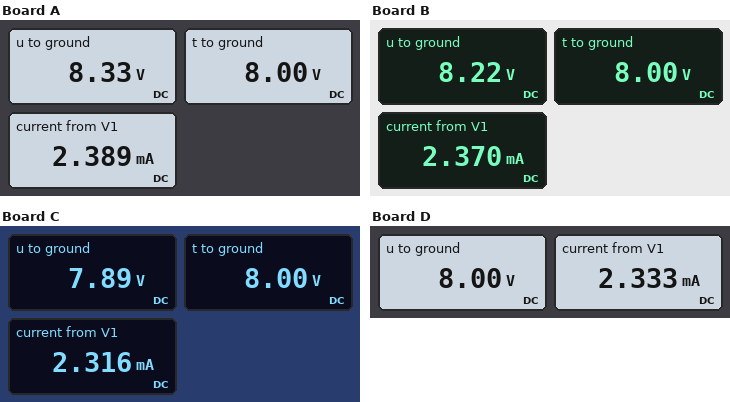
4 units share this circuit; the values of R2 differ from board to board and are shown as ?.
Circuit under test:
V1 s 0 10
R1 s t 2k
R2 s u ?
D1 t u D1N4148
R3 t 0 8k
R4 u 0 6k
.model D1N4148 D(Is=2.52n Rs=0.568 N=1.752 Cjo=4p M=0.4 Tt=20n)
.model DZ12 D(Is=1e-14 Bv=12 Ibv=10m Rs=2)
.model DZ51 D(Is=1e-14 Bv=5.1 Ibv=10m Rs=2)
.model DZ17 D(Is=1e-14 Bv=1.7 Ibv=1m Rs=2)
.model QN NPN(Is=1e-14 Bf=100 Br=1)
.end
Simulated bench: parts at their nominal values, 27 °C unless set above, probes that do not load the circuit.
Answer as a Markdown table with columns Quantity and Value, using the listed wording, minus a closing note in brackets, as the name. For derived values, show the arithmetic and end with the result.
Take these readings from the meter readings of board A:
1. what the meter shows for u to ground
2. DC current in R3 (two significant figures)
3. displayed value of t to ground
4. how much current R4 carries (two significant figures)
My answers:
| Quantity | Value |
|---|---|
| what the meter shows for u to ground | 8.33 V |
| DC current in R3 | (8 V) / 8 kΩ = 1.0 mA |
| displayed value of t to ground | 8.00 V |
| how much current R4 carries | (8.33 V) / 6 kΩ = 1.4 mA |
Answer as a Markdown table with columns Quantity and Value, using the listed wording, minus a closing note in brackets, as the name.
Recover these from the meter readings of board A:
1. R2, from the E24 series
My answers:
| Quantity | Value |
|---|---|
| R2, from the E24 series | 1.2 kΩ |
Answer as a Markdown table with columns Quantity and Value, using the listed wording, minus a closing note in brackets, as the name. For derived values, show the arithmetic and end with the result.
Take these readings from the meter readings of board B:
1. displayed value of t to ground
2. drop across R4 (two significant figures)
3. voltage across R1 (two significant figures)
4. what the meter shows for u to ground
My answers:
| Quantity | Value |
|---|---|
| displayed value of t to ground | 8.00 V |
| drop across R4 | 8.22 V = 8.2 V |
| voltage across R1 | 10 V - 8 V = 2.0 V |
| what the meter shows for u to ground | 8.22 V |
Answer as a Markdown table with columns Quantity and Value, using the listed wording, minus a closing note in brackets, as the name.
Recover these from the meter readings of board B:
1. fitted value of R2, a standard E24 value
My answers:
| Quantity | Value |
|---|---|
| fitted value of R2, a standard E24 value | 1.3 kΩ |
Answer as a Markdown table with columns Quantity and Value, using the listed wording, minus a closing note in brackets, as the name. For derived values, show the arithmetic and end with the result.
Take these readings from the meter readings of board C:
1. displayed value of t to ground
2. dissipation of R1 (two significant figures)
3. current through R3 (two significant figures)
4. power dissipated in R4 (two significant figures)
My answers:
| Quantity | Value |
|---|---|
| displayed value of t to ground | 8.00 V |
| dissipation of R1 | (10 V - 8 V)^2 / 2 kΩ = 2.0 mW |
| current through R3 | (8 V) / 8 kΩ = 1.0 mA |
| power dissipated in R4 | (7.89 V)^2 / 6 kΩ = 10 mW |
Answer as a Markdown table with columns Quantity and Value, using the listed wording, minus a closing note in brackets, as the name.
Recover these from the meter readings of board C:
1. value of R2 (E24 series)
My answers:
| Quantity | Value |
|---|---|
| value of R2 | 1.6 kΩ |
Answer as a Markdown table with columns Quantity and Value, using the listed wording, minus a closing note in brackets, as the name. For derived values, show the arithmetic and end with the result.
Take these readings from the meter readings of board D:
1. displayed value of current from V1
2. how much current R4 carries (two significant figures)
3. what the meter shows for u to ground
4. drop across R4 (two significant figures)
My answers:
| Quantity | Value |
|---|---|
| displayed value of current from V1 | 2.333 mA |
| how much current R4 carries | (8 V) / 6 kΩ = 1.3 mA |
| what the meter shows for u to ground | 8.00 V |
| drop across R4 | 8 V = 8.0 V |
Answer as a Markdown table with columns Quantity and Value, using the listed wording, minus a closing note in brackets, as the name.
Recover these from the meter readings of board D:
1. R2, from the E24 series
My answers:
| Quantity | Value |
|---|---|
| R2, from the E24 series | 1.5 kΩ |
